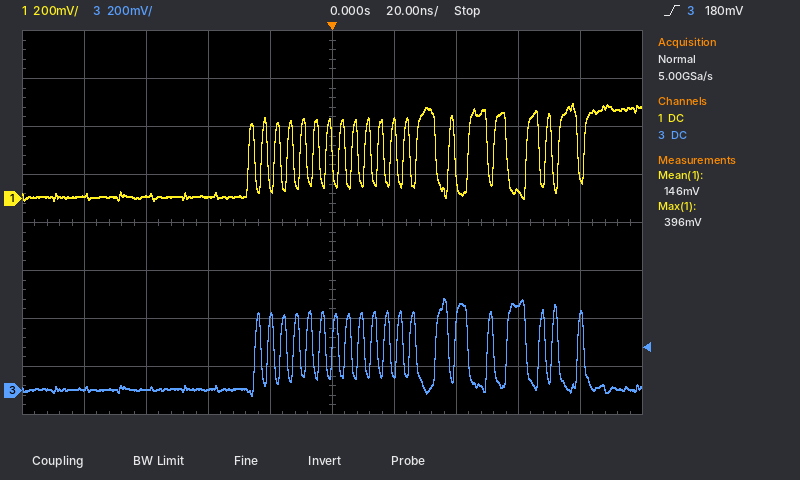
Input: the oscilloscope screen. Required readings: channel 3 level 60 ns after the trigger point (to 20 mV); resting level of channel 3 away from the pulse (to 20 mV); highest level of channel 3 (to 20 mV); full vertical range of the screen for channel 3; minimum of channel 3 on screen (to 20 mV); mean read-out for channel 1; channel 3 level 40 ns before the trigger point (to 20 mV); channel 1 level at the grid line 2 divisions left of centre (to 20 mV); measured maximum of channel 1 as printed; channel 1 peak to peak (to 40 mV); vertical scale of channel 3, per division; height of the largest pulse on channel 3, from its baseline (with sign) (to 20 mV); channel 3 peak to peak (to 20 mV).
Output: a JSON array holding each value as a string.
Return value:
["360 mV", "0 mV", "380 mV", "1.6 V", "-20 mV", "146 mV", "0 mV", "0 mV", "396 mV", "400 mV", "200 mV", "+380 mV", "400 mV"]
